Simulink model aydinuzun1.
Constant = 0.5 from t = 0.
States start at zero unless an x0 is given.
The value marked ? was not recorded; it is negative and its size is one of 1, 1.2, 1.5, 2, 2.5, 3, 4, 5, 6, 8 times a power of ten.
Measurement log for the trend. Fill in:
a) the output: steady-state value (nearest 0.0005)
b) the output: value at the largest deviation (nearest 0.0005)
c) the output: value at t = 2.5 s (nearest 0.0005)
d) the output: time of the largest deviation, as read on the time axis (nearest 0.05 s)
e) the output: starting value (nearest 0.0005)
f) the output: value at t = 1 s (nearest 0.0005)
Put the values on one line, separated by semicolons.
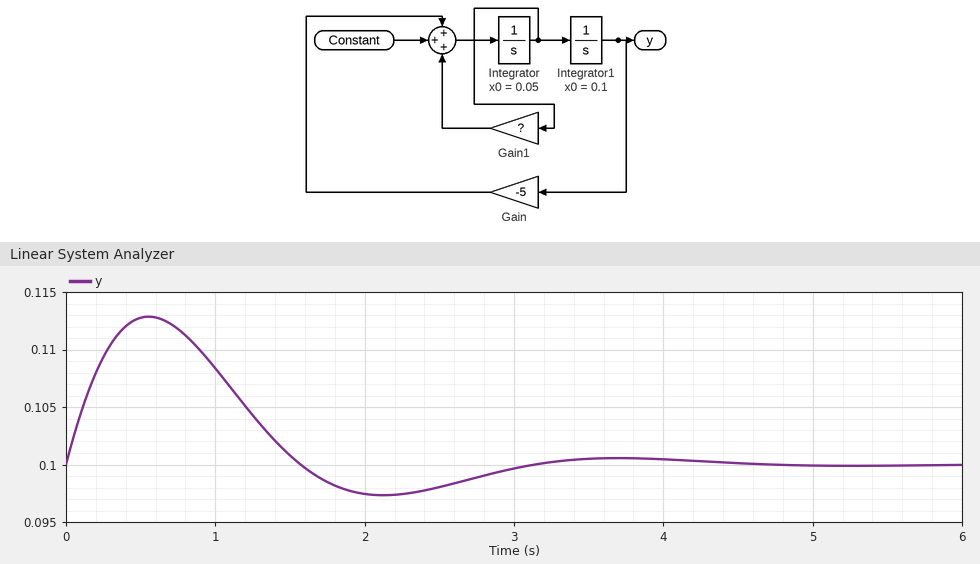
0.1000; 0.1130; 0.0980; 0.55 s; 0.1000; 0.1085
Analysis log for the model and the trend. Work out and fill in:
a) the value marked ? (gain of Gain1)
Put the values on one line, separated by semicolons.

-2
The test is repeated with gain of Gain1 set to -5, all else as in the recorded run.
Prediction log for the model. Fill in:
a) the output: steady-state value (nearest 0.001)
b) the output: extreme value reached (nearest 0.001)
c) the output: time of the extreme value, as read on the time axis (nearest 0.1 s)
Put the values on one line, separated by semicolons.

0.100; 0.108; 0.4 s
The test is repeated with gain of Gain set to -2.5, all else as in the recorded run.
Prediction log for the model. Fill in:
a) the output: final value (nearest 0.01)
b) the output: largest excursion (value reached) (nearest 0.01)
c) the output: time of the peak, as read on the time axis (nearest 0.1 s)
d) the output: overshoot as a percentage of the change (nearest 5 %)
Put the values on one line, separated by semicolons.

0.20; 0.21; 2.3 s; 10 %
